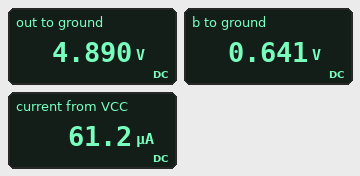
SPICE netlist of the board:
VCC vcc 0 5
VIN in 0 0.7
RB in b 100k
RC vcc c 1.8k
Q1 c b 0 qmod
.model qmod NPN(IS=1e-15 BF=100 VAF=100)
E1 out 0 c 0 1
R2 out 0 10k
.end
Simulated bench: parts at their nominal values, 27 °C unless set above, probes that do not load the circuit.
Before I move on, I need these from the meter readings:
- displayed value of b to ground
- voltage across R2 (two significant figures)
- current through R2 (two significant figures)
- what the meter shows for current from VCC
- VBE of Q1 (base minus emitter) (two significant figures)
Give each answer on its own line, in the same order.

0.641 V
4.9 V
490 µA
61.2 µA
640 mV
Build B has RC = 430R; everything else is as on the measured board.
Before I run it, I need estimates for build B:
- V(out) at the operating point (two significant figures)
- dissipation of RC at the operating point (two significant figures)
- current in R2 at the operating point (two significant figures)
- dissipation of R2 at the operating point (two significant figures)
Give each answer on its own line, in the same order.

5.0 V
1.6 µW
500 µA
2.5 mW
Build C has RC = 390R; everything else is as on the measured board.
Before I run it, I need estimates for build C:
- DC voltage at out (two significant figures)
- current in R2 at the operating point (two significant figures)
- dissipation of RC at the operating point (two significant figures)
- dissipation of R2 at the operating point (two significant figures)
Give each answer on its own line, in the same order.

5.0 V
500 µA
1.5 µW
2.5 mW
